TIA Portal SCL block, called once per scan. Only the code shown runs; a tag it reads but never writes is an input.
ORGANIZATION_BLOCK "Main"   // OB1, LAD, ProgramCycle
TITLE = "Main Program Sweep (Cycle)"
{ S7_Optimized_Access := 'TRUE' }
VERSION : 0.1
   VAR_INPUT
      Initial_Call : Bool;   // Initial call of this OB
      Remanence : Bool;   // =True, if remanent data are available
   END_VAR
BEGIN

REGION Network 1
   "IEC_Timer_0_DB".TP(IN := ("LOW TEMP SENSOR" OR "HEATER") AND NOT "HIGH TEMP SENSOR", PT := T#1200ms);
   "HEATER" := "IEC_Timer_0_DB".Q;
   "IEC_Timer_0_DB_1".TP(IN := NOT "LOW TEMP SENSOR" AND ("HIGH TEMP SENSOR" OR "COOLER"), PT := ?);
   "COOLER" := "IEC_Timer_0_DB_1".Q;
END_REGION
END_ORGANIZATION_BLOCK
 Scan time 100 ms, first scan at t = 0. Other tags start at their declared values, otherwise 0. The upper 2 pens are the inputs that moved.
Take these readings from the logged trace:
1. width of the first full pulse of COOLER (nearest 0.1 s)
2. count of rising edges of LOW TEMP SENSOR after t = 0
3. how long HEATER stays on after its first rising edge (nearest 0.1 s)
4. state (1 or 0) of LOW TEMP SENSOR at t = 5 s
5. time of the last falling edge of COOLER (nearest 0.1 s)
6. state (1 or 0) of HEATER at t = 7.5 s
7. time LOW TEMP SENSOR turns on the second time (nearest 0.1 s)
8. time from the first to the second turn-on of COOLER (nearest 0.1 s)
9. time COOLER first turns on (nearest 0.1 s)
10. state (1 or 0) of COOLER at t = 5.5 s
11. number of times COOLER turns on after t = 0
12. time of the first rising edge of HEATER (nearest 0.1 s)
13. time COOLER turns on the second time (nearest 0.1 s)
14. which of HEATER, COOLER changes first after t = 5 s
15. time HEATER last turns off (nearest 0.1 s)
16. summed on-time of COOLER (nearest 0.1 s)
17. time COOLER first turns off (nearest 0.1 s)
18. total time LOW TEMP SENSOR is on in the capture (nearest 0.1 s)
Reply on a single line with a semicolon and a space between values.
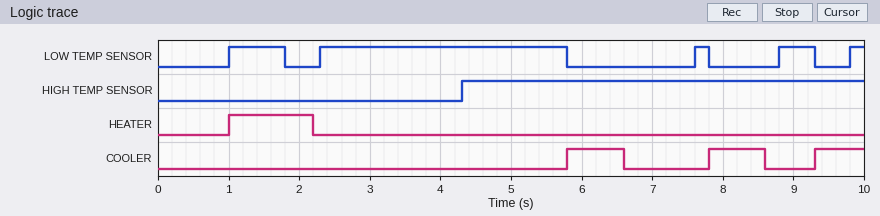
0.8 s; 5; 1.2 s; 1; 8.6 s; 0; 2.3 s; 2.0 s; 5.8 s; 0; 3; 1.0 s; 7.8 s; COOLER; 2.2 s; 2.3 s; 6.6 s; 5.2 s
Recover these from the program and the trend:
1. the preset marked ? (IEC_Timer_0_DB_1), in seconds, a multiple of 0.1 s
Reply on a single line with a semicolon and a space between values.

0.8 s
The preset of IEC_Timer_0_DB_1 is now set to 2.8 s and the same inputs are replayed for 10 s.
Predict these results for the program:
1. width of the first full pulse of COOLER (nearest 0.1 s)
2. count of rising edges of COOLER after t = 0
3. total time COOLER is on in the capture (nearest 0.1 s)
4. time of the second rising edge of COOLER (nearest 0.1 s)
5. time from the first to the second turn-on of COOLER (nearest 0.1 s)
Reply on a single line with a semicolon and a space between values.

2.8 s; 2; 3.5 s; 9.3 s; 3.5 s
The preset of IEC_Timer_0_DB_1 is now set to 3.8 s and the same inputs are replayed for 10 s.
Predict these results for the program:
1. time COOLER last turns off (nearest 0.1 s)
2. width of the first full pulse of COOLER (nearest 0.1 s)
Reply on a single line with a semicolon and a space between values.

9.6 s; 3.8 s
